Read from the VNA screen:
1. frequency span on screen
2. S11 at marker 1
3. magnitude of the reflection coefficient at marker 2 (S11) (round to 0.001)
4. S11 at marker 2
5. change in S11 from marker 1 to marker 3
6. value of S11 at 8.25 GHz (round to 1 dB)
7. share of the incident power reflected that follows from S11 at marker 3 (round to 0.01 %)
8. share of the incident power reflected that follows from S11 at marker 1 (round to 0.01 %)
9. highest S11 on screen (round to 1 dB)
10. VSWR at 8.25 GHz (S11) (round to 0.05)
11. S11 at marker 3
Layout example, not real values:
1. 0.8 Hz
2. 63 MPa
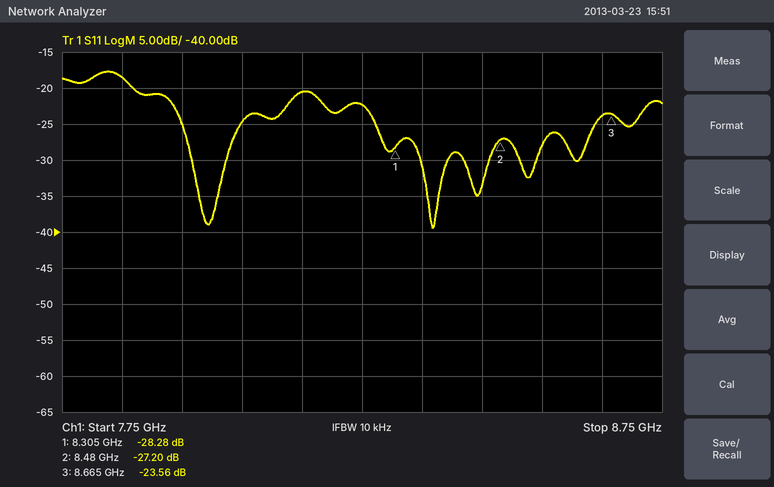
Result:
1. 1 GHz
2. -28.28 dB
3. 0.044
4. -27.20 dB
5. 4.72 dB
6. -22 dB
7. 0.44 %
8. 0.15 %
9. -18 dB
10. 1.15
11. -23.56 dB
